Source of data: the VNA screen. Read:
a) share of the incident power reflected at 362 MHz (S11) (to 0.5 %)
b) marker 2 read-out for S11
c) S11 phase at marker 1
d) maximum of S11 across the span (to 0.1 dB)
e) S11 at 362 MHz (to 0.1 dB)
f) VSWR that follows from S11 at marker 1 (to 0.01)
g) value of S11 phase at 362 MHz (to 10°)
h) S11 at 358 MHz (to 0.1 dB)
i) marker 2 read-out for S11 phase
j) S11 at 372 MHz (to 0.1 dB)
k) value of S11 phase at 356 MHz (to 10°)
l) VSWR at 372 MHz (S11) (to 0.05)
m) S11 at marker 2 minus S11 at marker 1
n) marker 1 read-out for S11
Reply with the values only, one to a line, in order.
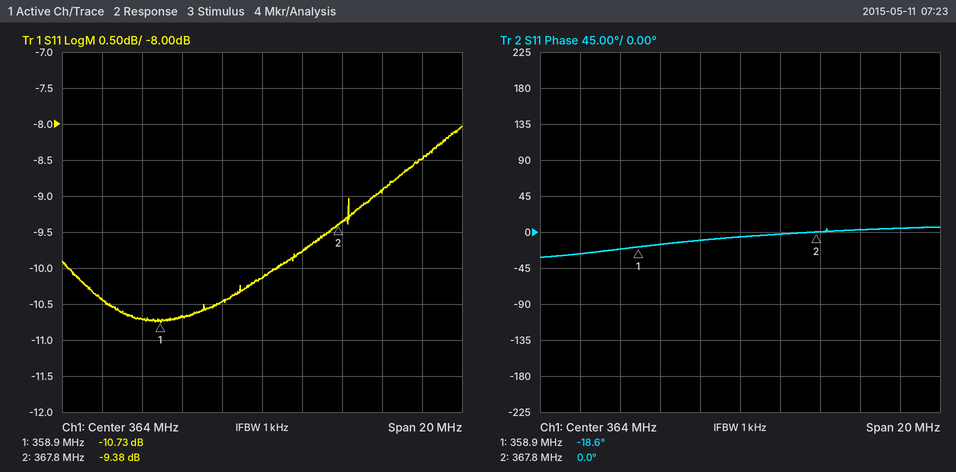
9.0 %
-9.38 dB
-18.6°
-8.0 dB
-10.5 dB
1.82
-10°
-10.7 dB
0.0°
-8.5 dB
-30°
2.20
1.35 dB
-10.73 dB
